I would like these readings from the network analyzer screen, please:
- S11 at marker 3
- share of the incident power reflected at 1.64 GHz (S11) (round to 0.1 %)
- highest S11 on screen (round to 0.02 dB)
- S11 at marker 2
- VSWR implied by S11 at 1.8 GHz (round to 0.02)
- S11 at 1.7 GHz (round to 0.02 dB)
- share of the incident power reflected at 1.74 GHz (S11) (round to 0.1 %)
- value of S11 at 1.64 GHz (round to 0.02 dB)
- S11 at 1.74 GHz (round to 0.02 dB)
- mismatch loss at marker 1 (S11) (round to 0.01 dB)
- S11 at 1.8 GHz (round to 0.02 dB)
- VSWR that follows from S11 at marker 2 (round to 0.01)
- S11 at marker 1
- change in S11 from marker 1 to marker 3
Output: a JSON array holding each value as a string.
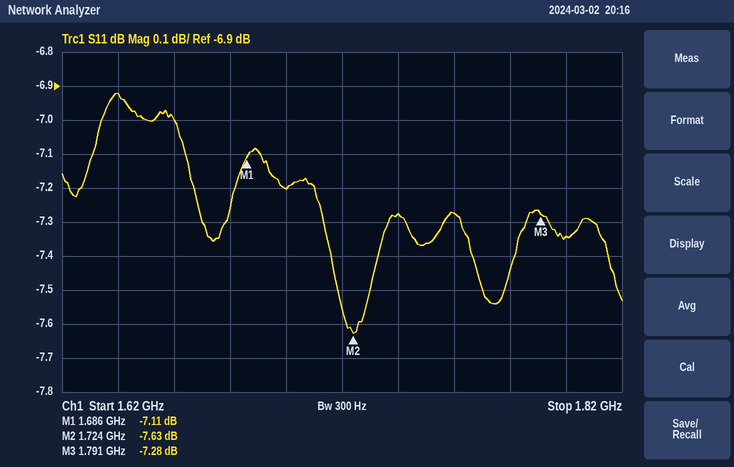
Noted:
["-7.28 dB", "20.3 %", "-6.92 dB", "-7.63 dB", "2.50", "-7.20 dB", "18.7 %", "-6.92 dB", "-7.28 dB", "0.94 dB", "-7.34 dB", "2.42", "-7.11 dB", "-0.17 dB"]
